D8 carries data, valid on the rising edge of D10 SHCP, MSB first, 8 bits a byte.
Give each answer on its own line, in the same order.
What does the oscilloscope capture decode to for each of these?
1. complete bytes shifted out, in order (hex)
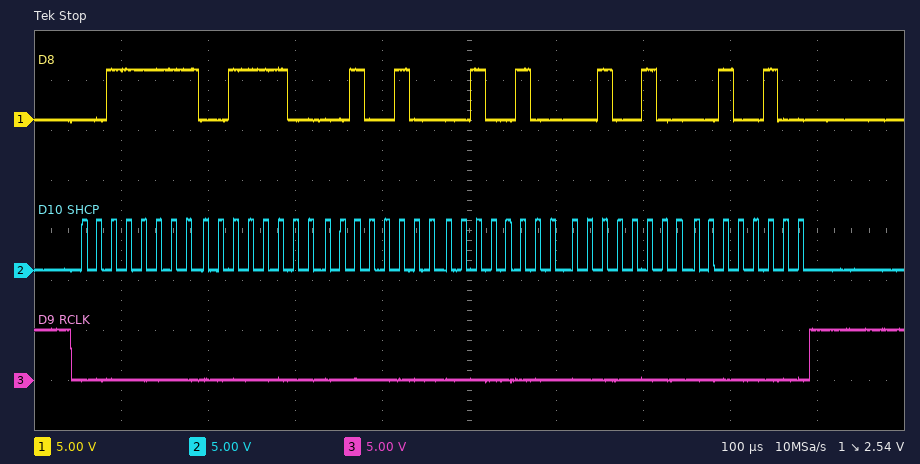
3F 3C 24 24 24 24
